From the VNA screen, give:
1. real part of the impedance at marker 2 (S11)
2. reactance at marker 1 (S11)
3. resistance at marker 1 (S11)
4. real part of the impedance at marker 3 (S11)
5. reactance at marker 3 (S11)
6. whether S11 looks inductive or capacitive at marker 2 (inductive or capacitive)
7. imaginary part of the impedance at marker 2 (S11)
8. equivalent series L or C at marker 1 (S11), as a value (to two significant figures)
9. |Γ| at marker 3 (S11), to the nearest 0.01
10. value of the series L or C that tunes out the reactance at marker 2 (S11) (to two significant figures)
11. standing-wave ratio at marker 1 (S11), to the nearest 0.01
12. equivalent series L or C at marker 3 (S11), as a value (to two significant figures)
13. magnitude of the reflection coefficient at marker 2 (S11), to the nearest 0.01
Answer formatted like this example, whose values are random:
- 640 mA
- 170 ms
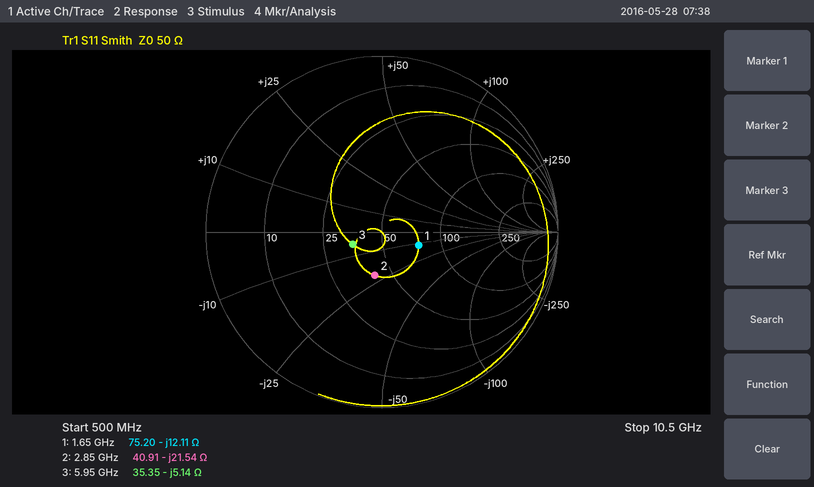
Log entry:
- 40.91 Ω
- -12.11 Ω
- 75.20 Ω
- 35.35 Ω
- -5.14 Ω
- capacitive
- -21.54 Ω
- 8.0 pF
- 0.18
- 1.2 nH
- 1.57
- 5.2 pF
- 0.25
